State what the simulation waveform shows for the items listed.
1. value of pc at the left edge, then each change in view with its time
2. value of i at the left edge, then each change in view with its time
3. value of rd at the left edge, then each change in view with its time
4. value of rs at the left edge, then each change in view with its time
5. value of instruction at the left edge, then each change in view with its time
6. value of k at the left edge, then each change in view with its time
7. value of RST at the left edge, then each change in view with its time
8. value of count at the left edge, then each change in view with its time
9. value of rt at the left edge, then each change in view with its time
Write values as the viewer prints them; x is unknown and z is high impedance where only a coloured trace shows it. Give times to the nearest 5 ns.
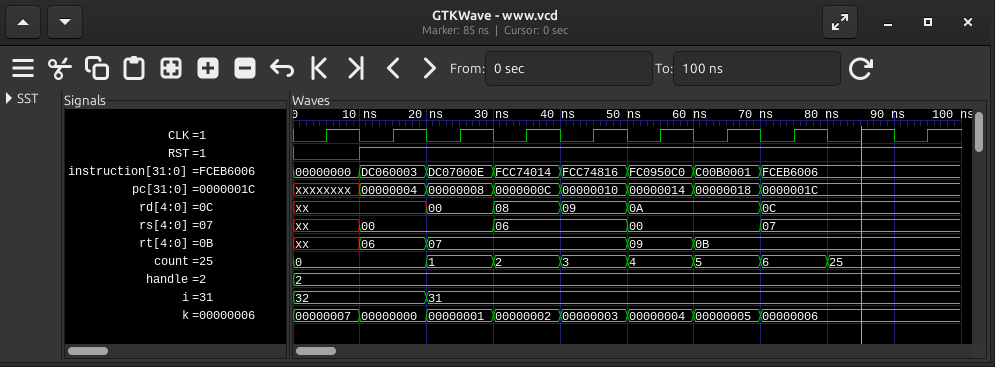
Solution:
xxxxxxxx, 00000004 at 10 ns, 00000008 at 20 ns, 0000000C at 30 ns, 00000010 at 40 ns, 00000014 at 50 ns, 00000018 at 60 ns, 0000001C at 70 ns
32, 31 at 20 ns
xx, 00 at 20 ns, 08 at 30 ns, 09 at 40 ns, 0A at 50 ns, 0C at 70 ns
xx, 00 at 10 ns, 06 at 30 ns, 00 at 50 ns, 07 at 70 ns
00000000, DC060003 at 10 ns, DC07000E at 20 ns, FCC74014 at 30 ns, FCC74816 at 40 ns, FC0950C0 at 50 ns, C00B0001 at 60 ns, FCEB6006 at 70 ns
00000007, 00000000 at 10 ns, 00000001 at 20 ns, 00000002 at 30 ns, 00000003 at 40 ns, 00000004 at 50 ns, 00000005 at 60 ns, 00000006 at 70 ns
0, 1 at 10 ns
0, 1 at 20 ns, 2 at 30 ns, 3 at 40 ns, 4 at 50 ns, 5 at 60 ns, 6 at 70 ns, 25 at 80 ns
xx, 06 at 10 ns, 07 at 20 ns, 09 at 50 ns, 0B at 60 ns
